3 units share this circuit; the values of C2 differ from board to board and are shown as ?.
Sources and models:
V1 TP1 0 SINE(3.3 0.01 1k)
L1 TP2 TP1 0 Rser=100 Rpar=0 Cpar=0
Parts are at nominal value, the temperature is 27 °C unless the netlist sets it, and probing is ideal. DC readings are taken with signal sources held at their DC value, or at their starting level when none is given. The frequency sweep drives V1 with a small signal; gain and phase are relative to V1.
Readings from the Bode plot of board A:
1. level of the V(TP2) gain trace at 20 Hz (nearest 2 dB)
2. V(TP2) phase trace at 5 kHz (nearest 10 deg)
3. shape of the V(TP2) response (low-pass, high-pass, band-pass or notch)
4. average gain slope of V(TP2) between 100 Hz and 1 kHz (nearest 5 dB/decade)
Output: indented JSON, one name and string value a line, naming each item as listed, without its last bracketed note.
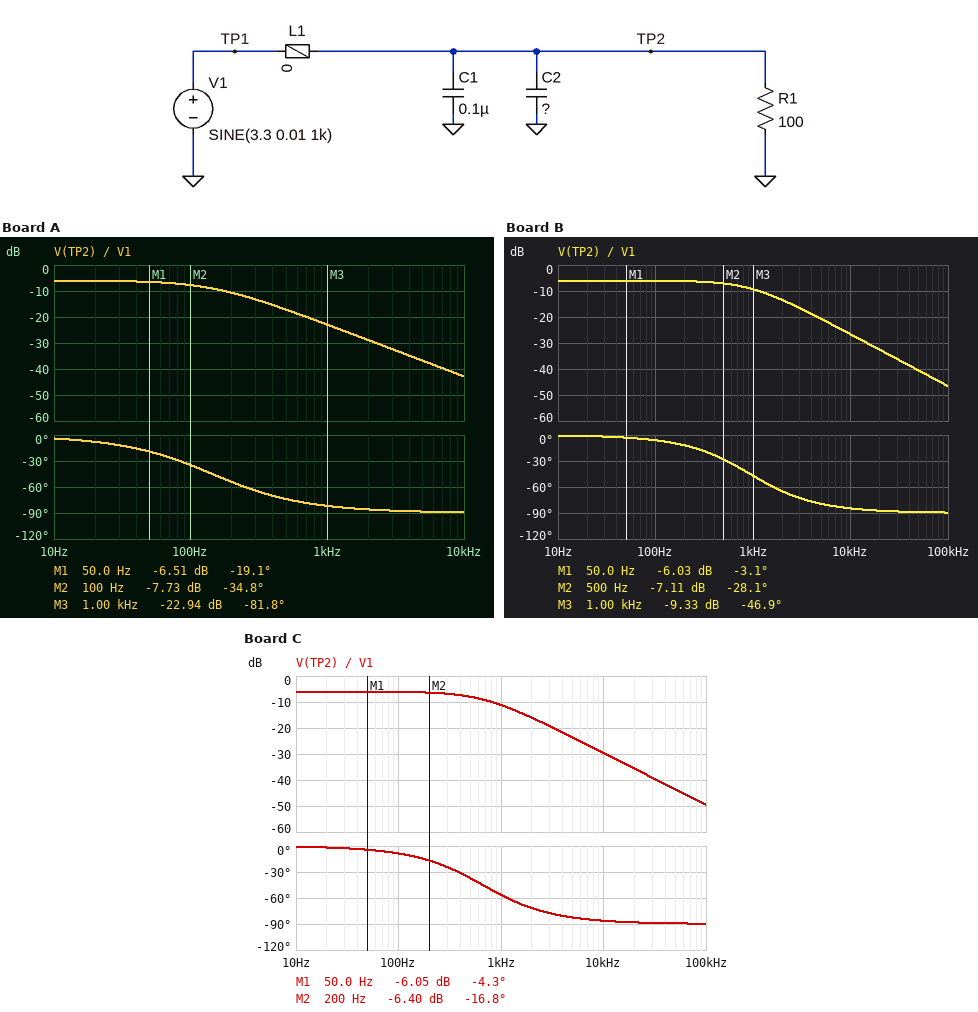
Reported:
{
  "level of the V(TP2) gain trace at 20 Hz": "-6 dB",
  "V(TP2) phase trace at 5 kHz": "-90 deg",
  "shape of the V(TP2) response": "low-pass",
  "average gain slope of V(TP2) between 100 Hz and 1 kHz": "-15 dB/decade"
}
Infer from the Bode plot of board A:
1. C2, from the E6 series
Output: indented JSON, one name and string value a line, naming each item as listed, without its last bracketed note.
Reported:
{
  "C2, from the E6 series": "22 µF"
}
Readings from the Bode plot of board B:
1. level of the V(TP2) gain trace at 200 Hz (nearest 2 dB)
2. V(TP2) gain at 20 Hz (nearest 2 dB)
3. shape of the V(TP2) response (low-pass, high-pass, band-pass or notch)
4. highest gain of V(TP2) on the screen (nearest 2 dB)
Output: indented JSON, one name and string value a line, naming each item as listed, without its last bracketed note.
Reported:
{
  "level of the V(TP2) gain trace at 200 Hz": "-6 dB",
  "V(TP2) gain at 20 Hz": "-6 dB",
  "shape of the V(TP2) response": "low-pass",
  "highest gain of V(TP2) on the screen": "-6 dB"
}
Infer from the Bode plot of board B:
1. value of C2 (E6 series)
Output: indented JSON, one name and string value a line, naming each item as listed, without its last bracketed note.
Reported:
{
  "value of C2": "3.3 µF"
}
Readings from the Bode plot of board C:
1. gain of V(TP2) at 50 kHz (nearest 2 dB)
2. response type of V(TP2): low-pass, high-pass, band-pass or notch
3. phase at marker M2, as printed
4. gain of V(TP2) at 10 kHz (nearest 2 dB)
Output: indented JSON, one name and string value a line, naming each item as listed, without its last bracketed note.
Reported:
{
  "gain of V(TP2) at 50 kHz": "-44 dB",
  "response type of V(TP2): low-pass, high-pass, band-pass or notch": "low-pass",
  "phase at marker M2, as printed": "-16.8 deg",
  "gain of V(TP2) at 10 kHz": "-30 dB"
}
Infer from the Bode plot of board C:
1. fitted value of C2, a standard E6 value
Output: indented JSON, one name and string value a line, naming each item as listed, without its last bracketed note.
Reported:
{
  "fitted value of C2, a standard E6 value": "4.7 µF"
}
